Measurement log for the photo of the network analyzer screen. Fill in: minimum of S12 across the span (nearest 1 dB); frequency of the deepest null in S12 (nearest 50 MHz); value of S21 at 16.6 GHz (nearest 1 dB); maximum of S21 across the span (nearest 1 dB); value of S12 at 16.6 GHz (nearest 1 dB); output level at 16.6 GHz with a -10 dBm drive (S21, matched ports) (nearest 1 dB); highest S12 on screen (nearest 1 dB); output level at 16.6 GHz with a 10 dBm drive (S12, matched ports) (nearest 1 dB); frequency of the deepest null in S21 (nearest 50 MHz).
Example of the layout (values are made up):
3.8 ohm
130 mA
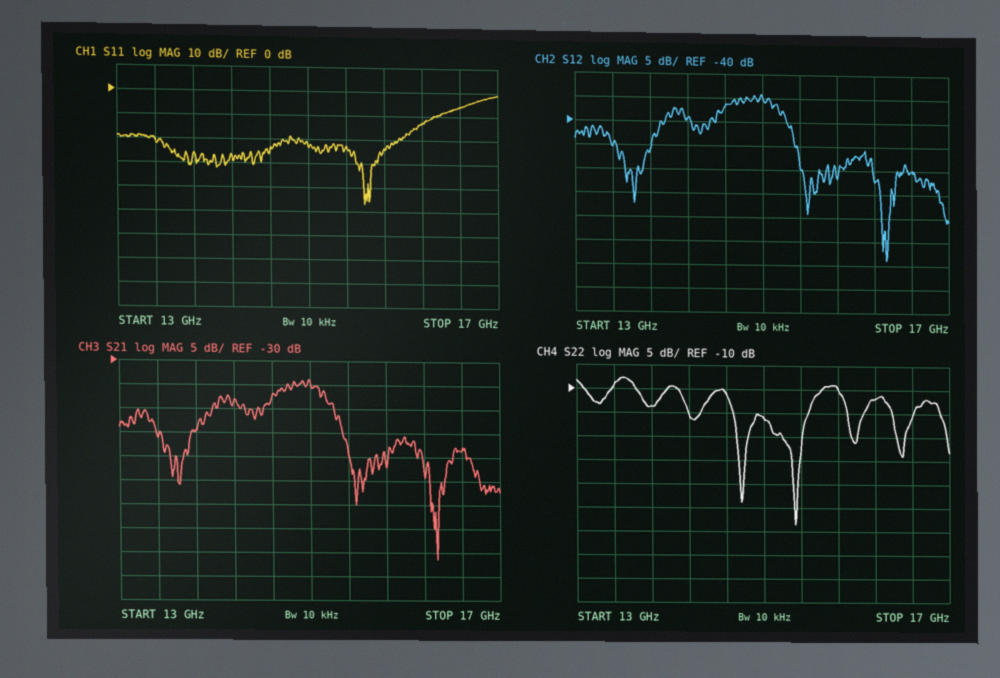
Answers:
-69 dB
16.35 GHz
-48 dB
-34 dB
-50 dB
-58 dBm
-34 dB
-40 dBm
16.35 GHz
